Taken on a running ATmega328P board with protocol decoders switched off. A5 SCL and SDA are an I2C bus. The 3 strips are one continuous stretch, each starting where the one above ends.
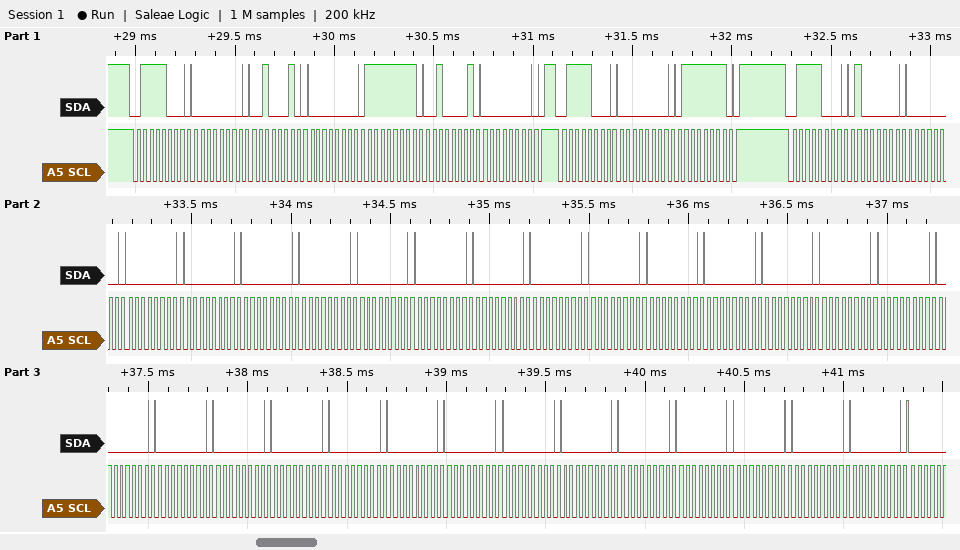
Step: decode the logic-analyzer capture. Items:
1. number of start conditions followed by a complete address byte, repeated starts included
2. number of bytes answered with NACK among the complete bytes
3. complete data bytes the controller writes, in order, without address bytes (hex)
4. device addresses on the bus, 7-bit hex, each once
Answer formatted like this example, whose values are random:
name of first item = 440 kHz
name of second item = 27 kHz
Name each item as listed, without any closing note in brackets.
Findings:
number of start conditions followed by a complete address byte, repeated starts included = 3
number of bytes answered with NACK among the complete bytes = 0
complete data bytes the controller writes, in order, without address bytes = 00 22 00 FF 21 00 00 7F 40 00 00 00 00 00 00 00 00 00 00 00 00 00 00 00 00 00 00 00 00 00 00 00 00 00 00 00 00 00
device addresses on the bus, 7-bit hex, each once = 0x3C
